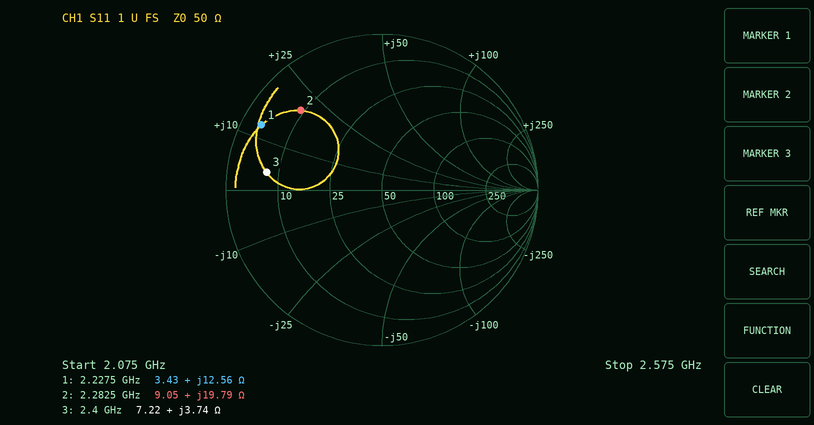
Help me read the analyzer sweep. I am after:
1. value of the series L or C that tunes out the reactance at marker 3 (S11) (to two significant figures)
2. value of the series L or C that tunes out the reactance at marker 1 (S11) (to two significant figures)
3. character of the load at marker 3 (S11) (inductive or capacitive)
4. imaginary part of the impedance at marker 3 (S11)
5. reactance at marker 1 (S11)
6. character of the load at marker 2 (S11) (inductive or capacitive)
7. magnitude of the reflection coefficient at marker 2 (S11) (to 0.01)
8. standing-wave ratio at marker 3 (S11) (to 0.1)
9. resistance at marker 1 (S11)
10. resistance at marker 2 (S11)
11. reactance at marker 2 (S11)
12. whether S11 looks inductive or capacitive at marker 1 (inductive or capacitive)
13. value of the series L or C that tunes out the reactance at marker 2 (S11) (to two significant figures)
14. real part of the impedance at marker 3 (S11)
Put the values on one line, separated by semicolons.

18 pF; 5.7 pF; inductive; +3.74 Ω; +12.56 Ω; inductive; 0.73; 7.0; 3.43 Ω; 9.05 Ω; +19.79 Ω; inductive; 3.5 pF; 7.22 Ω
